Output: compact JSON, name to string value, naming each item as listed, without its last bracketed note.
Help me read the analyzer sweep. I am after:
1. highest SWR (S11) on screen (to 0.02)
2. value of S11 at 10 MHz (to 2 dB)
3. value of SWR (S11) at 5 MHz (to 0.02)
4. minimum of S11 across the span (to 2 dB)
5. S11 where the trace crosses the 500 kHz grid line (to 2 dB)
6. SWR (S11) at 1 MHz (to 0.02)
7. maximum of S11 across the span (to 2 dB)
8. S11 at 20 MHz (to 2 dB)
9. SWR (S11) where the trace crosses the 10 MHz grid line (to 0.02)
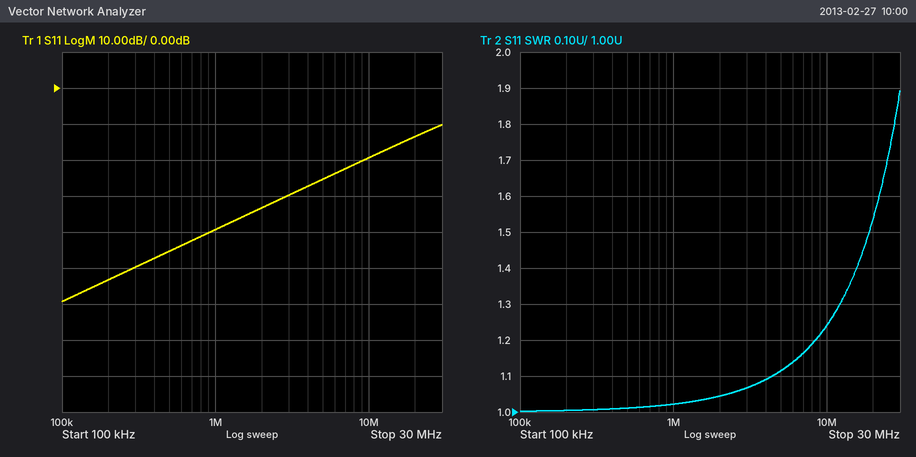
{"highest SWR (S11) on screen": "1.90", "value of S11 at 10 MHz": "-20 dB", "value of SWR (S11) at 5 MHz": "1.12", "minimum of S11 across the span": "-60 dB", "S11 where the trace crosses the 500 kHz grid line": "-46 dB", "SWR (S11) at 1 MHz": "1.02", "maximum of S11 across the span": "-10 dB", "S11 at 20 MHz": "-14 dB", "SWR (S11) where the trace crosses the 10 MHz grid line": "1.24"}
